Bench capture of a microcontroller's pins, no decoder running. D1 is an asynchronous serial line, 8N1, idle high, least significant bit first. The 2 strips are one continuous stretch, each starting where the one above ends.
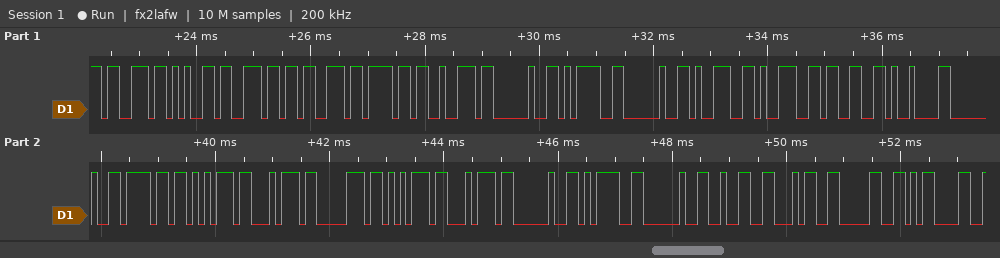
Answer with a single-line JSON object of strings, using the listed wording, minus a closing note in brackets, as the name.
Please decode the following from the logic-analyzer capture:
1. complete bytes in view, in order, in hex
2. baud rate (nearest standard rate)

{"complete bytes in view, in order, in hex": "73 65 6E 73 6F 72 20 3D 20 39 39 33 09 20 6F 75 74 70 75 74 20 3D 20 32 34 30 0D", "baud rate": "9600 baud"}
